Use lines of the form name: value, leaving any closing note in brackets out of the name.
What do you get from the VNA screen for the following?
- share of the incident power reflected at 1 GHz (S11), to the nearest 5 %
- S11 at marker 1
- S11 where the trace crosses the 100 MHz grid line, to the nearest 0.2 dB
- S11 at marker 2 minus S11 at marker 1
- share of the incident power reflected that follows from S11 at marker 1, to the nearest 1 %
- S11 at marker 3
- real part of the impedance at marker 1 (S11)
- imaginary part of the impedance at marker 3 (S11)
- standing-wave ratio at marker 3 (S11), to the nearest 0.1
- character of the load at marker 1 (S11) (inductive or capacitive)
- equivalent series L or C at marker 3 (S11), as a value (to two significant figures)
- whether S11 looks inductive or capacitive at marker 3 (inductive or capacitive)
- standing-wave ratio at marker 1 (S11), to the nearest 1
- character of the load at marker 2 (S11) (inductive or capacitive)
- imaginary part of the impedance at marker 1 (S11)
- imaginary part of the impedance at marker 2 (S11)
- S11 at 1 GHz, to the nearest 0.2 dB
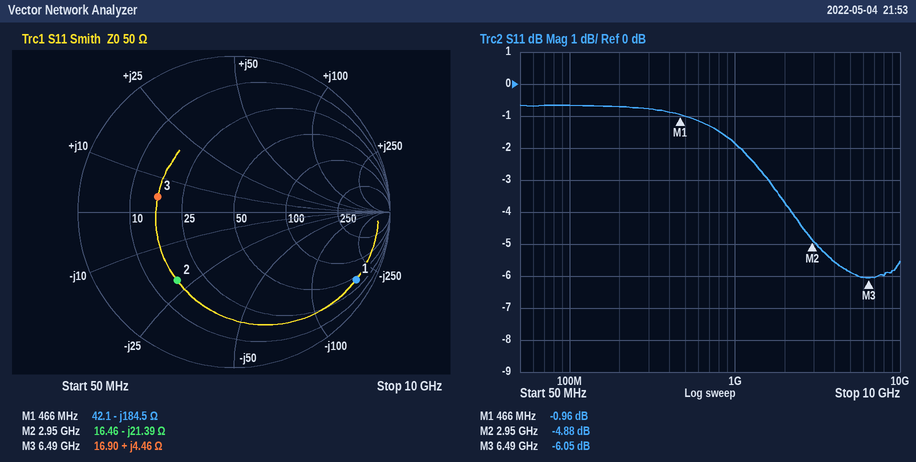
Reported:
share of the incident power reflected at 1 GHz (S11), to the nearest 5 %: 65 %
S11 at marker 1: -0.96 dB
S11 where the trace crosses the 100 MHz grid line, to the nearest 0.2 dB: -0.6 dB
S11 at marker 2 minus S11 at marker 1: -3.92 dB
share of the incident power reflected that follows from S11 at marker 1, to the nearest 1 %: 80 %
S11 at marker 3: -6.05 dB
real part of the impedance at marker 1: 42.1 Ω
imaginary part of the impedance at marker 3: +4.46 Ω
standing-wave ratio at marker 3 (S11), to the nearest 0.1: 3.0
character of the load at marker 1 (S11): capacitive
equivalent series L or C at marker 3 (S11), as a value: 110 pH
whether S11 looks inductive or capacitive at marker 3: inductive
standing-wave ratio at marker 1 (S11), to the nearest 1: 18
character of the load at marker 2 (S11): capacitive
imaginary part of the impedance at marker 1: -184.5 Ω
imaginary part of the impedance at marker 2: -21.39 Ω
S11 at 1 GHz, to the nearest 0.2 dB: -1.8 dB
